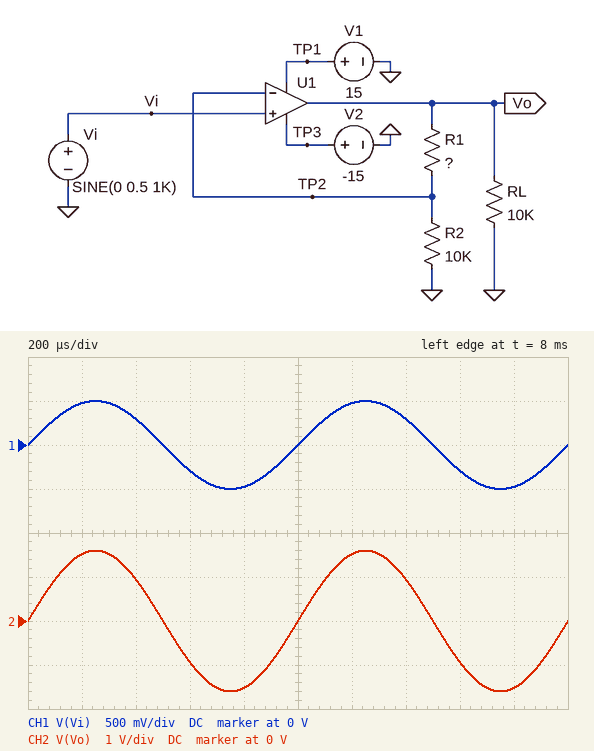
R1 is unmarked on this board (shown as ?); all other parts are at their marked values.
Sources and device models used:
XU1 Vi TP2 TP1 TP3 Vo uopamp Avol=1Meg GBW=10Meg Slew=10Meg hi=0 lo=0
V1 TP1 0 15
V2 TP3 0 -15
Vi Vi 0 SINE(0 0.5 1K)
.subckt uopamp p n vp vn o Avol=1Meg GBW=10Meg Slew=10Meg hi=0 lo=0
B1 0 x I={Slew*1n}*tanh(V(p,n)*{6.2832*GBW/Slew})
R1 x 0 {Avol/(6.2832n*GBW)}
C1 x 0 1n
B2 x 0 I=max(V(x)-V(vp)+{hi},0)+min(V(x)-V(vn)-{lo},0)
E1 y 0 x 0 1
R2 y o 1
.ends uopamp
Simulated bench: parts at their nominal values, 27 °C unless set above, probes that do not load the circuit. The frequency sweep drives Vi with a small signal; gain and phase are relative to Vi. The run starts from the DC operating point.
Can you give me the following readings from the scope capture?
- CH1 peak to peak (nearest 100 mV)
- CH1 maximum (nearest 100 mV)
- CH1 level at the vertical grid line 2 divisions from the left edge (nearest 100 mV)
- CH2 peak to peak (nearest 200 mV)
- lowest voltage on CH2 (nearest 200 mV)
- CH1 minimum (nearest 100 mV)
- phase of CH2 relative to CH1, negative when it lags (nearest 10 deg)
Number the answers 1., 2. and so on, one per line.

1. 1.0 V
2. 500 mV
3. 300 mV
4. 3.2 V
5. -1.6 V
6. -500 mV
7. 0 deg
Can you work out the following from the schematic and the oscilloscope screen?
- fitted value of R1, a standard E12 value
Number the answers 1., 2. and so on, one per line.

1. 22 kΩ
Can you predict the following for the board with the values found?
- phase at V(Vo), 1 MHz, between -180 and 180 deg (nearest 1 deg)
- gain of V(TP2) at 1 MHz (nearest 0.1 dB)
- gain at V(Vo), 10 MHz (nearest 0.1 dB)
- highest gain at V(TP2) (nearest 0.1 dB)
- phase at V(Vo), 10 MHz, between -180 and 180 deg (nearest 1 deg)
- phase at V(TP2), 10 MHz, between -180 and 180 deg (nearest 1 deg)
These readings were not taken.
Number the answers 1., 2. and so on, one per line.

1. -18 deg
2. -0.4 dB
3. -0.4 dB
4. 0 dB
5. -73 deg
6. -73 deg
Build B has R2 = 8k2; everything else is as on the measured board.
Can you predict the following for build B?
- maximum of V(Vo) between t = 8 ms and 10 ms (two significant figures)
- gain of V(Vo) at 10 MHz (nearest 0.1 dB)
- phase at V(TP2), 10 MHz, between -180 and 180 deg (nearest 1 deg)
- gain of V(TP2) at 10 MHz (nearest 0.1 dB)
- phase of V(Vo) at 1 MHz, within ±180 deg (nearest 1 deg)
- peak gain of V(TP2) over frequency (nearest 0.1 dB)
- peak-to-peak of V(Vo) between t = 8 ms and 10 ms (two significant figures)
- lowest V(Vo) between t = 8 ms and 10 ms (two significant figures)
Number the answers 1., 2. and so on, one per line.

1. 1.8 V
2. -0.3 dB
3. -75 deg
4. -11.6 dB
5. -20 deg
6. 0 dB
7. 3.7 V
8. -1.8 V
